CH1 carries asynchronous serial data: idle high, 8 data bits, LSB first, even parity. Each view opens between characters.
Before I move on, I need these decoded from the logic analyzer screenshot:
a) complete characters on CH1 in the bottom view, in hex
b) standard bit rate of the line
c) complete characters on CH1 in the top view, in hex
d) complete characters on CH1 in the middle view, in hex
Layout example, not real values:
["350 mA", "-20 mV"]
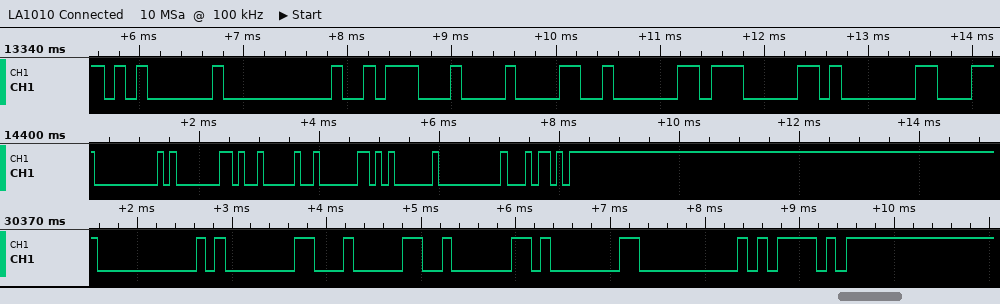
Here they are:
["00, 01, 04, 02, 01, 00, BD", "9600 baud", "05, 00, 3A, 08, 02, 07, 01", "00, 01, 09, 02, 05, 00, B4"]
